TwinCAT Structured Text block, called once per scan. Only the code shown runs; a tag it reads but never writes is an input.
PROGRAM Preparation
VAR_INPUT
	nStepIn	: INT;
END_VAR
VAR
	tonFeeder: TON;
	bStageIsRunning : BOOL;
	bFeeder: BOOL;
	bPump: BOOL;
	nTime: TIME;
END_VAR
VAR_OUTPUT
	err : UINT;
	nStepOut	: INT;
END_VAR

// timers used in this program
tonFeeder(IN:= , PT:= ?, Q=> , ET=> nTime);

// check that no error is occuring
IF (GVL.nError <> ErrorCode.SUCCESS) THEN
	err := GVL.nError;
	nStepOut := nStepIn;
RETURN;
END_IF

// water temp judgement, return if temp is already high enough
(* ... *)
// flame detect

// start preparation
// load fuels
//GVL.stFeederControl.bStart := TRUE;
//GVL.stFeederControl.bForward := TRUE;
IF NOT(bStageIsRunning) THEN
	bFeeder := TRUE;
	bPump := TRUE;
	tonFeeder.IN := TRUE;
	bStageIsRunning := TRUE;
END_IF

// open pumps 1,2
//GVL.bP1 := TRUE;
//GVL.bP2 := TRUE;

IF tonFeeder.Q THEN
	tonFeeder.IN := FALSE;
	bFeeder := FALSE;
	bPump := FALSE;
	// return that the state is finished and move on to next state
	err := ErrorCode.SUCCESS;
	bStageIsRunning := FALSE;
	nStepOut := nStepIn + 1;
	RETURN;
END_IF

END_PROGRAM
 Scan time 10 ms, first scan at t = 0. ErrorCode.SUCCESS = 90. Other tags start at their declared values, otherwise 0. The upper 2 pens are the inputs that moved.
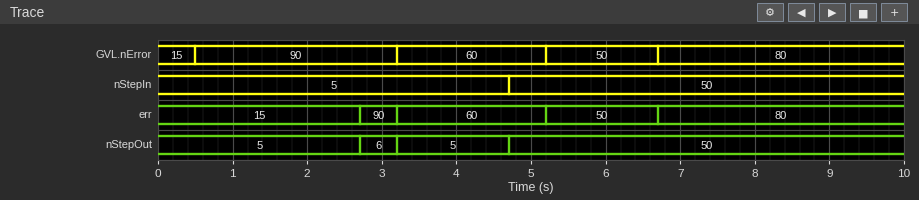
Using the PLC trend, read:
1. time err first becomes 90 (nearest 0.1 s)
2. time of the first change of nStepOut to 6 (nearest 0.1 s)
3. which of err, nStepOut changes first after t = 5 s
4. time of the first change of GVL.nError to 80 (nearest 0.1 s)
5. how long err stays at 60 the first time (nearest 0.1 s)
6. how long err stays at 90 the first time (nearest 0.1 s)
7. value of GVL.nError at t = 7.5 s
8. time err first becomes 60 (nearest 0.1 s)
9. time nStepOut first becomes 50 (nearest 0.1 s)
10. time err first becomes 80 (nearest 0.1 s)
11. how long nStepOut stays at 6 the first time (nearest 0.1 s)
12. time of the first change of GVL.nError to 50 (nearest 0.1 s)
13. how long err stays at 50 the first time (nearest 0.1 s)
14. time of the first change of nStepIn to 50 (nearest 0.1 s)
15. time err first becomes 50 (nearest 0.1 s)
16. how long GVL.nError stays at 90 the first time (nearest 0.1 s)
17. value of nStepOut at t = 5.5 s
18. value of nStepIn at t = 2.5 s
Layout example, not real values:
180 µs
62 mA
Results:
2.7 s
2.7 s
err
6.7 s
2.0 s
0.5 s
80
3.2 s
4.7 s
6.7 s
0.5 s
5.2 s
1.5 s
4.7 s
5.2 s
2.7 s
50
5
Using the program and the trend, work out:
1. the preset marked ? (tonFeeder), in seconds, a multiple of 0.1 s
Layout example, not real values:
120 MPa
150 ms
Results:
2.2 s
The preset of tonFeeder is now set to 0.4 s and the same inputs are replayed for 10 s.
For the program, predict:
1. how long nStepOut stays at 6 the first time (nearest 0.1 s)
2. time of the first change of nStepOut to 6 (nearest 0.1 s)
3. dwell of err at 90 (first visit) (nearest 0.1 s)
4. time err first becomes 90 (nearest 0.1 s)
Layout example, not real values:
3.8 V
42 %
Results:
2.3 s
0.9 s
2.3 s
0.9 s
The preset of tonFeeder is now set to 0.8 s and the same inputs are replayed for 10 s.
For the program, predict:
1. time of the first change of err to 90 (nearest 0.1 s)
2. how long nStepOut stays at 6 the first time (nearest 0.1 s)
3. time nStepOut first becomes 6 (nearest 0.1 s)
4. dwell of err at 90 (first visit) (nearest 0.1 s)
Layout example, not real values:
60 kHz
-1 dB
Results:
1.3 s
1.9 s
1.3 s
1.9 s
